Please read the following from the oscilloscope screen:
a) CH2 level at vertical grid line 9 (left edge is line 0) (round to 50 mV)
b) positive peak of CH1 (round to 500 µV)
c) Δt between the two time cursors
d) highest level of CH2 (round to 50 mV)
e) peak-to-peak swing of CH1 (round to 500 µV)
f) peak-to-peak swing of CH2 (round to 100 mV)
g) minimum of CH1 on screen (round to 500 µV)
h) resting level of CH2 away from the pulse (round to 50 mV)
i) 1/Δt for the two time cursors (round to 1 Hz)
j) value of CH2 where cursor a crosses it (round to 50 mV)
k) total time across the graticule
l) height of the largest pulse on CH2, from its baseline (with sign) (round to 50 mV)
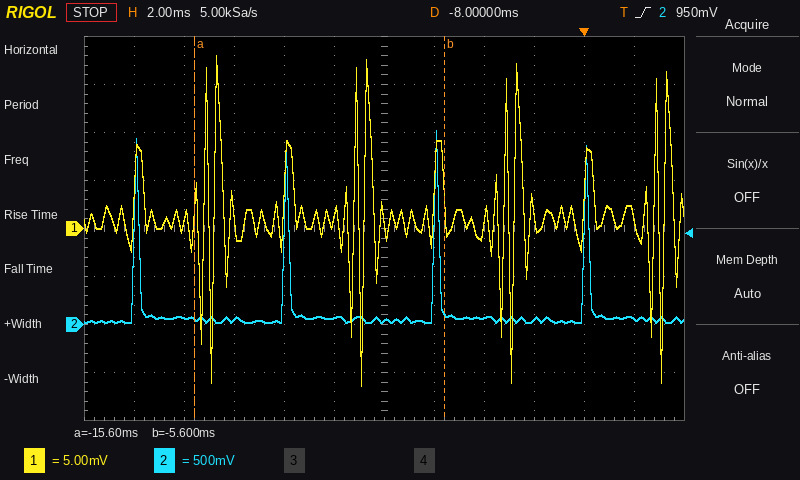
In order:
50 mV
18.0 mV
10.0 ms
2.00 V
34.5 mV
2.00 V
-16.5 mV
50 mV
100 Hz
50 mV
24 ms
+1.95 V
